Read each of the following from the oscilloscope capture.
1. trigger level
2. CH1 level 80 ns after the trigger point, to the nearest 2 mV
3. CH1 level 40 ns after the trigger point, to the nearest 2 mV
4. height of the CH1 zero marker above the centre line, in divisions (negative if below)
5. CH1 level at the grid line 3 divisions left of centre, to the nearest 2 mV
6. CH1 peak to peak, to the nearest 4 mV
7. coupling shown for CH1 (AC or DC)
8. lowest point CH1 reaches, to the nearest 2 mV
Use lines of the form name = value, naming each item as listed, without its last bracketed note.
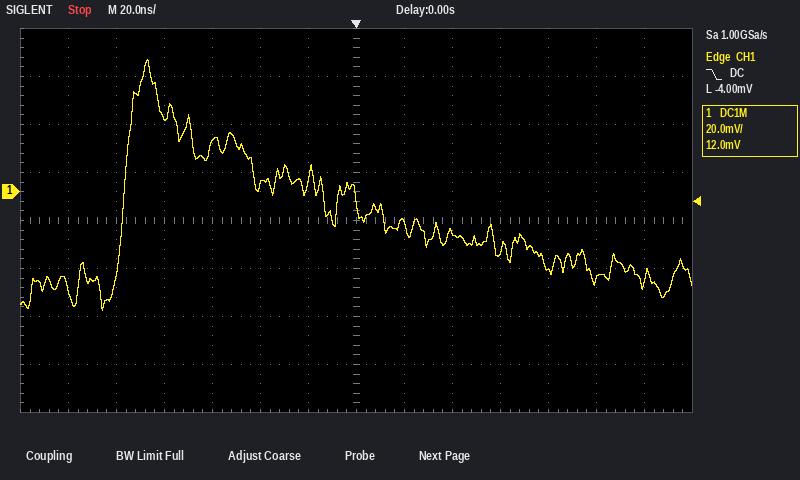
trigger level = -4.00 mV
CH1 level 80 ns after the trigger point, to the nearest 2 mV = -32 mV
CH1 level 40 ns after the trigger point, to the nearest 2 mV = -16 mV
height of the CH1 zero marker above the centre line, in divisions = +0.6 div
CH1 level at the grid line 3 divisions left of centre, to the nearest 2 mV = 20 mV
CH1 peak to peak, to the nearest 4 mV = 104 mV
coupling shown for CH1 = DC
lowest point CH1 reaches, to the nearest 2 mV = -50 mV
